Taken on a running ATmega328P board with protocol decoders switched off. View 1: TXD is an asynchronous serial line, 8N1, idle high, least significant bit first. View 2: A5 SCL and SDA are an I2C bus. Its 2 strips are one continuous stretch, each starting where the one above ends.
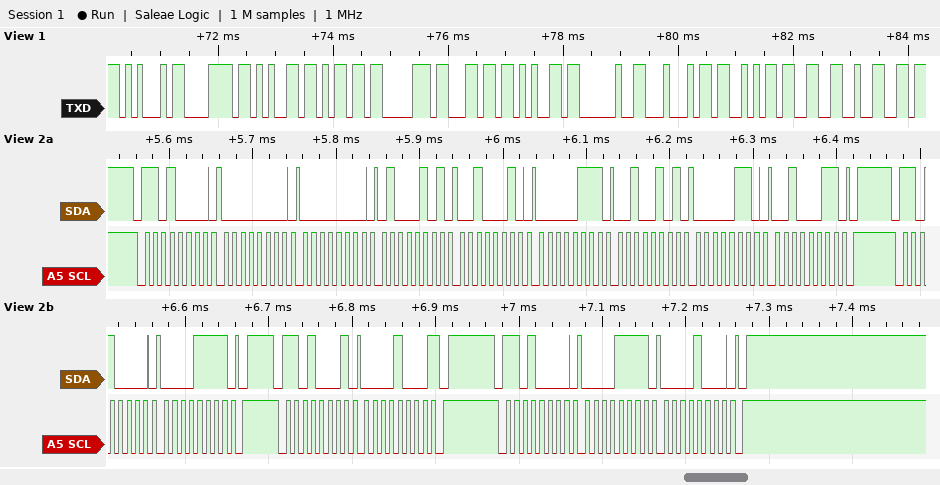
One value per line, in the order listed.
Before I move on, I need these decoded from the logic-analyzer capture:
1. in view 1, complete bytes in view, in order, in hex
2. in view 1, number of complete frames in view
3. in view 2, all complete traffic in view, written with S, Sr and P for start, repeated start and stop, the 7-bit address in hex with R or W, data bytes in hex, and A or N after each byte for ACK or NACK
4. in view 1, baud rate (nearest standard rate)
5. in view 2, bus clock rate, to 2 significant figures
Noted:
45 78 65 6D 70 6C 65 20 44 53 33 32
12
S 68W A 00 A 00 A 45 A 22 A 07 A 25 A 06 A 23 A P S 68W A 0F A P S 68R A 08 N P S 68W A 0F A 08 A P
9600 baud
100 kHz
